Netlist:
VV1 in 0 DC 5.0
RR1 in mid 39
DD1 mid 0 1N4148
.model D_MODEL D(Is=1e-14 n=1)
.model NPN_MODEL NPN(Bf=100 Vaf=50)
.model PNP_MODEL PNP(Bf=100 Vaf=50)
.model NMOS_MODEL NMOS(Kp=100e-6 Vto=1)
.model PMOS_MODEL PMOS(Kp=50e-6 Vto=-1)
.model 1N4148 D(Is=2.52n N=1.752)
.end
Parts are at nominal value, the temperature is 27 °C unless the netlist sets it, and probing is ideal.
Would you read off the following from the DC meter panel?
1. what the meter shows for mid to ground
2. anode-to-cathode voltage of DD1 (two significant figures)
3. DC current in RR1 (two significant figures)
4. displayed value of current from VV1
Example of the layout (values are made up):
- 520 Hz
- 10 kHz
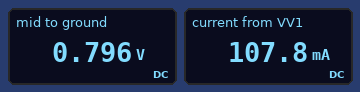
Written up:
- 0.796 V
- 800 mV
- 110 mA
- 107.8 mA
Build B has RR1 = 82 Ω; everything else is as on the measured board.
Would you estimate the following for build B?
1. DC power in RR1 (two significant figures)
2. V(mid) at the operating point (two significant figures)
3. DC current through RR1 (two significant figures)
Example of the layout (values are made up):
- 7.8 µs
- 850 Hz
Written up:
- 220 mW
- 760 mV
- 52 mA
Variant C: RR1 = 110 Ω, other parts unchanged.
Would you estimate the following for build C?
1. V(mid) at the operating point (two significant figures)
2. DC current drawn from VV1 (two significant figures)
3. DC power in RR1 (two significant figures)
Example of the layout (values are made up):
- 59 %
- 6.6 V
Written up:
- 750 mV
- 39 mA
- 160 mW
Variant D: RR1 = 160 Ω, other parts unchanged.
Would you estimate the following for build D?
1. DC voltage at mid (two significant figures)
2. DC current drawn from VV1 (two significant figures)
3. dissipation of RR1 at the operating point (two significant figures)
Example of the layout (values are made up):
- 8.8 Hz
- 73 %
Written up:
- 730 mV
- 27 mA
- 110 mW
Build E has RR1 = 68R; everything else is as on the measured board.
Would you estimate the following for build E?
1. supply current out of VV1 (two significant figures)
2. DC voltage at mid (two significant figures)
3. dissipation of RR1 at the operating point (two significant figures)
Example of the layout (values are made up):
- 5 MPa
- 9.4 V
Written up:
- 62 mA
- 770 mV
- 260 mW
